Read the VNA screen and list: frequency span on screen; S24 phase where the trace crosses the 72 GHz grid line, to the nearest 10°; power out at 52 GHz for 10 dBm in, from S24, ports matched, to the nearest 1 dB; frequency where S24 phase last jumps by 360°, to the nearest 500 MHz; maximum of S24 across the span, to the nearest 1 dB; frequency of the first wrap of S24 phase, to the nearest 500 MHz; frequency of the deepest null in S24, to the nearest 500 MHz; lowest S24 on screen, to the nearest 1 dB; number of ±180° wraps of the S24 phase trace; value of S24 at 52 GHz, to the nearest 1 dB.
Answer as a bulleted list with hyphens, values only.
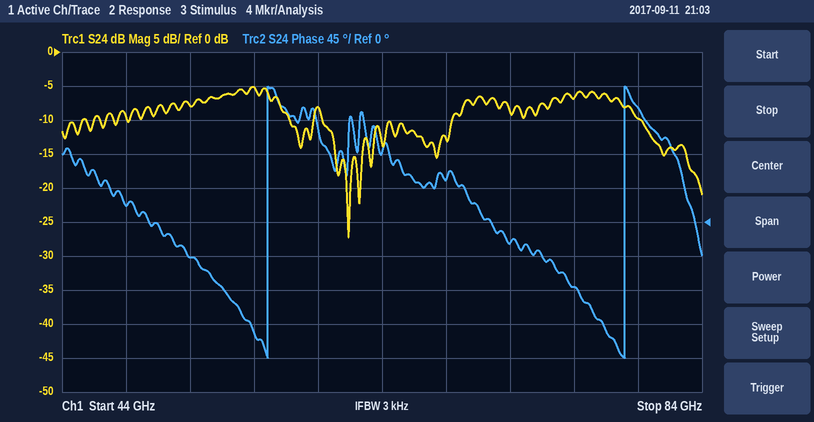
- 40 GHz
- -30°
- 2 dBm
- 79.0 GHz
- -5 dB
- 57.0 GHz
- 62.0 GHz
- -27 dB
- 2
- -8 dB
